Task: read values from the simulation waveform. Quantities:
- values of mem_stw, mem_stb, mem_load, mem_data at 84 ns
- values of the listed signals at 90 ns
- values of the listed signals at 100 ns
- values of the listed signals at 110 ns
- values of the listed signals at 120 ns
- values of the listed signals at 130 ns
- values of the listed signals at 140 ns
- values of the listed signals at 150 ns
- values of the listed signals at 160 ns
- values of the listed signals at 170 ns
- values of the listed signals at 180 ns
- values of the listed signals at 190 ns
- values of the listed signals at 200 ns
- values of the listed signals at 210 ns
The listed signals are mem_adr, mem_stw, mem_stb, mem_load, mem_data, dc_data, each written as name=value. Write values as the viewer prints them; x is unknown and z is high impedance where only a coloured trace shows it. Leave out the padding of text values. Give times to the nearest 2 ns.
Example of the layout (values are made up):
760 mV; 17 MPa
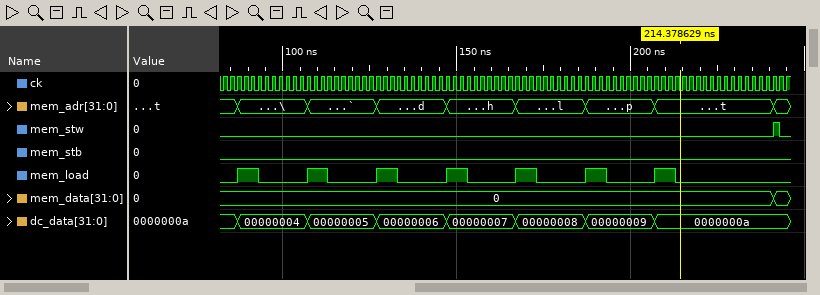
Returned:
mem_stw=0, mem_stb=0, mem_load=0, mem_data=0; mem_adr=\, mem_stw=0, mem_stb=0, mem_load=1, mem_data=0, dc_data=00000004; mem_adr=\, mem_stw=0, mem_stb=0, mem_load=0, mem_data=0, dc_data=00000004; mem_adr=`, mem_stw=0, mem_stb=0, mem_load=1, mem_data=0, dc_data=00000005; mem_adr=`, mem_stw=0, mem_stb=0, mem_load=0, mem_data=0, dc_data=00000005; mem_adr=d, mem_stw=0, mem_stb=0, mem_load=1, mem_data=0, dc_data=00000006; mem_adr=d, mem_stw=0, mem_stb=0, mem_load=0, mem_data=0, dc_data=00000006; mem_adr=h, mem_stw=0, mem_stb=0, mem_load=1, mem_data=0, dc_data=00000007; mem_adr=h, mem_stw=0, mem_stb=0, mem_load=0, mem_data=0, dc_data=00000007; mem_adr=l, mem_stw=0, mem_stb=0, mem_load=1, mem_data=0, dc_data=00000008; mem_adr=l, mem_stw=0, mem_stb=0, mem_load=0, mem_data=0, dc_data=00000008; mem_adr=p, mem_stw=0, mem_stb=0, mem_load=1, mem_data=0, dc_data=00000009; mem_adr=p, mem_stw=0, mem_stb=0, mem_load=0, mem_data=0, dc_data=00000009; mem_adr=t, mem_stw=0, mem_stb=0, mem_load=1, mem_data=0, dc_data=0000000a
